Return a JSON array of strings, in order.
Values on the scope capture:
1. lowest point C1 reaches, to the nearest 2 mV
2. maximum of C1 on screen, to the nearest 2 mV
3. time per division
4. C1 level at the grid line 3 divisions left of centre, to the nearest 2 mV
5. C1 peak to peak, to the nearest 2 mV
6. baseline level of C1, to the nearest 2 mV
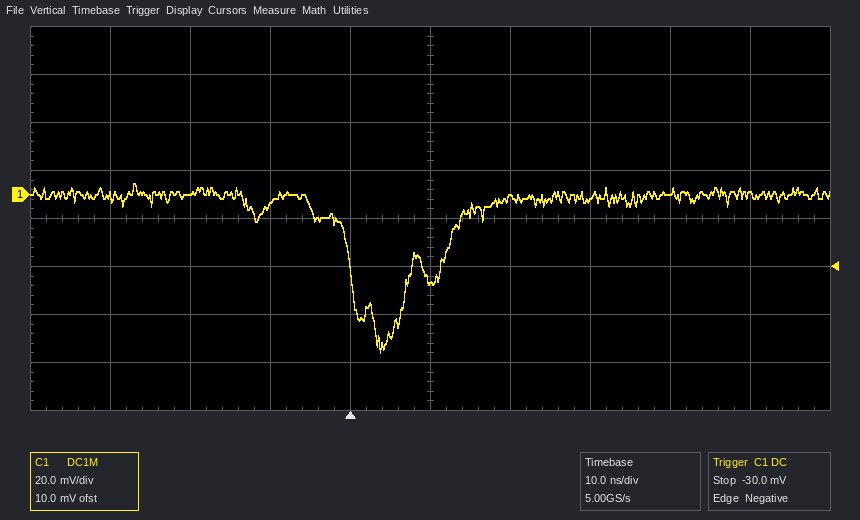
["-66 mV", "4 mV", "10 ns", "0 mV", "70 mV", "0 mV"]
